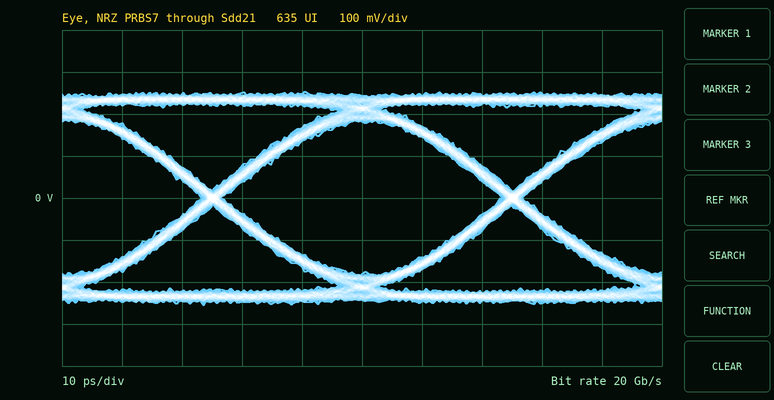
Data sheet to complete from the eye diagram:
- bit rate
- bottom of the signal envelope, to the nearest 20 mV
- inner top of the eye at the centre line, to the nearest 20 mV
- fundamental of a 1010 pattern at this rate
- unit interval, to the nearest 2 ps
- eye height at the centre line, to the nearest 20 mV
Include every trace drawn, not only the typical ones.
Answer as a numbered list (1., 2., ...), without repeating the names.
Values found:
1. 20 Gb/s
2. -260 mV
3. 180 mV
4. 10 GHz
5. 50 ps
6. 360 mV
